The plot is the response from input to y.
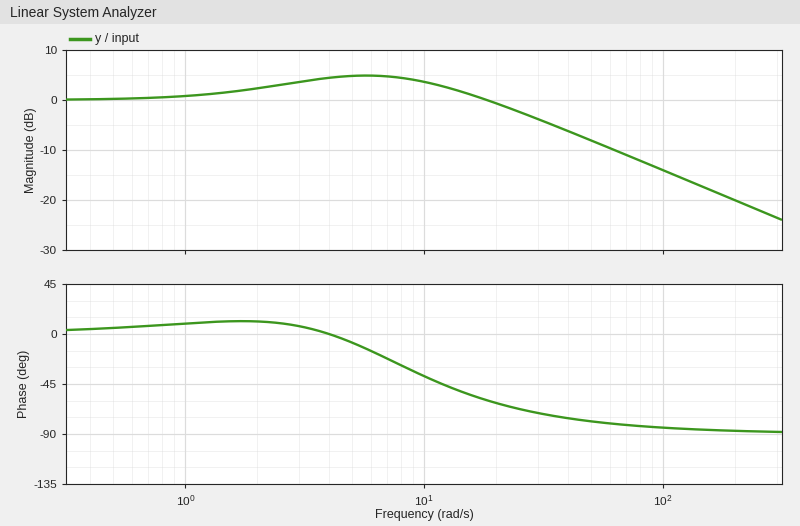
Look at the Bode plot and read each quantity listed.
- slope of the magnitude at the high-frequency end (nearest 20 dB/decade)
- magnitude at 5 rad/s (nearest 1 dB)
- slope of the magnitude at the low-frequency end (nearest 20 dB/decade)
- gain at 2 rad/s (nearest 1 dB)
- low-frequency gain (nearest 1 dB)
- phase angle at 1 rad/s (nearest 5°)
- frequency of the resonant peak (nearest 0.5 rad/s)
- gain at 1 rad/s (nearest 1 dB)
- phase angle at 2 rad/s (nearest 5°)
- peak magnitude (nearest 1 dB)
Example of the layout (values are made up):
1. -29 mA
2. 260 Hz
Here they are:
1. -20 dB/decade
2. 5 dB
3. 0 dB/decade
4. 2 dB
5. 0 dB
6. 10°
7. 5.5 rad/s
8. 1 dB
9. 10°
10. 5 dB
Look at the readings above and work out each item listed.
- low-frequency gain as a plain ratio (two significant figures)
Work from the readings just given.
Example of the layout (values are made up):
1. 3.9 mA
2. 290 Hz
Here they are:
1. 1.0
